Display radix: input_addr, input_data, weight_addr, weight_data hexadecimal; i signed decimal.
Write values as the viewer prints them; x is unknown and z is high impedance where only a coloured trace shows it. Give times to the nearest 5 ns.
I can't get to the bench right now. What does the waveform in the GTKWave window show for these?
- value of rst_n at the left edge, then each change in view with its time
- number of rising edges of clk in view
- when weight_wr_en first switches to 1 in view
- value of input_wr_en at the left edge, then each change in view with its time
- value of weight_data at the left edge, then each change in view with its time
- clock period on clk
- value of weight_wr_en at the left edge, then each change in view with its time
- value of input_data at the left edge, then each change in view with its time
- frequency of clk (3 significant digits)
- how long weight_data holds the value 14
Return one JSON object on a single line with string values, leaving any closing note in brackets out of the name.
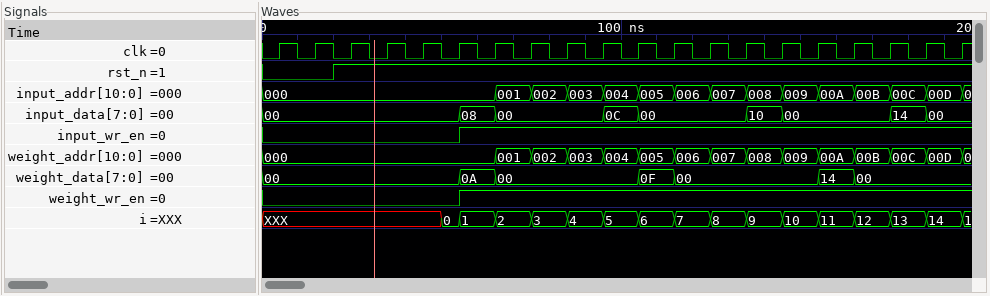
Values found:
{"value of rst_n at the left edge, then each change in view with its time": "0, 1 at 20 ns", "number of rising edges of clk in view": "20", "when weight_wr_en first switches to 1 in view": "55 ns", "value of input_wr_en at the left edge, then each change in view with its time": "0, 1 at 55 ns", "value of weight_data at the left edge, then each change in view with its time": "00, 0A at 55 ns, 00 at 65 ns, 0F at 105 ns, 00 at 115 ns, 14 at 155 ns, 00 at 165 ns", "clock period on clk": "10 ns", "value of weight_wr_en at the left edge, then each change in view with its time": "0, 1 at 55 ns", "value of input_data at the left edge, then each change in view with its time": "00, 08 at 55 ns, 00 at 65 ns, 0C at 95 ns, 00 at 105 ns, 10 at 135 ns, 00 at 145 ns, 14 at 175 ns, 00 at 185 ns", "frequency of clk": "100 MHz", "how long weight_data holds the value 14": "10 ns"}
